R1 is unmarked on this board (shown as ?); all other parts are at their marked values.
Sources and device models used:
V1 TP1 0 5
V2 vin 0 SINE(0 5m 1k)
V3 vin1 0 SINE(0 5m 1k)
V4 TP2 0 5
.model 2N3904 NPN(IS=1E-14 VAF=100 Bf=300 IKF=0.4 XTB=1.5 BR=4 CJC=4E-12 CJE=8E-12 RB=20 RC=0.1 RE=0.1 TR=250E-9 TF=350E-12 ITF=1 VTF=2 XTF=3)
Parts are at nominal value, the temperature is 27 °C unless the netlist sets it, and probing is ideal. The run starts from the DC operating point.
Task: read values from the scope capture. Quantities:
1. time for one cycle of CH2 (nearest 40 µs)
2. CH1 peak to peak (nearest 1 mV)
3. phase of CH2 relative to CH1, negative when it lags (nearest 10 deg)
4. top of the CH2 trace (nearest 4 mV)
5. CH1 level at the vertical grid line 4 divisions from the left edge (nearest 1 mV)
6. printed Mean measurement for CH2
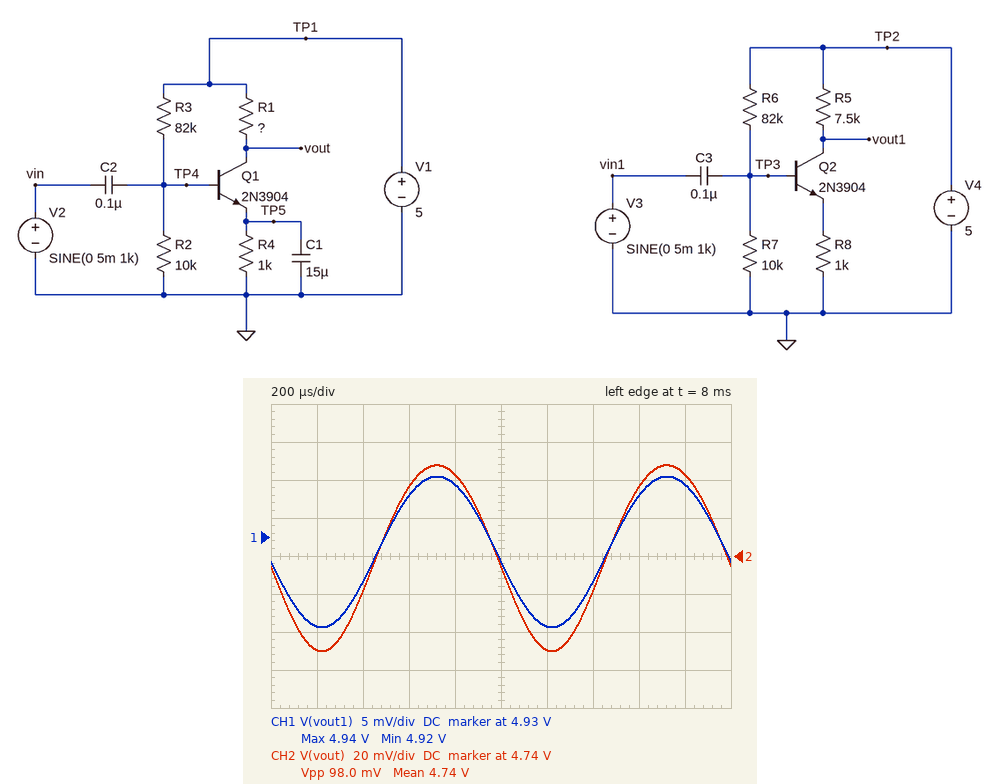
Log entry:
1.00 ms
20 mV
0 deg
4.788 V
4.937 V
4.74 V
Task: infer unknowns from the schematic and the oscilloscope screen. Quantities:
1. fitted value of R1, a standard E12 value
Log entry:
27 kΩ
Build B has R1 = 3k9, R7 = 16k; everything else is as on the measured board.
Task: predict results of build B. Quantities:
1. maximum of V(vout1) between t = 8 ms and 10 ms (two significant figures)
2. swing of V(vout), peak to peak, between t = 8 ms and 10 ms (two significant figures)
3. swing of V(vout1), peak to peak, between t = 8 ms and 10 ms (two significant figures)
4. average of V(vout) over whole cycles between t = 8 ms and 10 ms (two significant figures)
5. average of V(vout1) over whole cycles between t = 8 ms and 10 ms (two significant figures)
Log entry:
3.6 V
14 mV
65 mV
5.0 V
3.5 V
